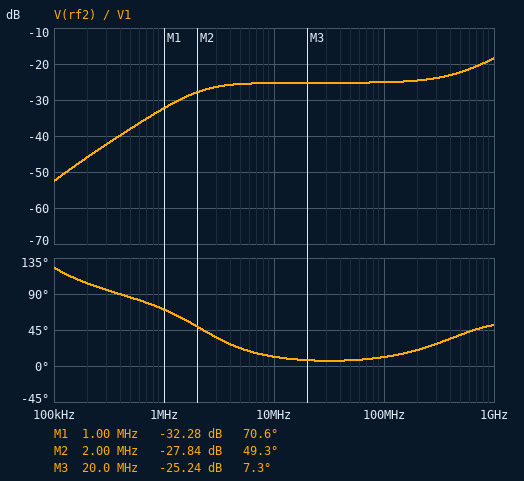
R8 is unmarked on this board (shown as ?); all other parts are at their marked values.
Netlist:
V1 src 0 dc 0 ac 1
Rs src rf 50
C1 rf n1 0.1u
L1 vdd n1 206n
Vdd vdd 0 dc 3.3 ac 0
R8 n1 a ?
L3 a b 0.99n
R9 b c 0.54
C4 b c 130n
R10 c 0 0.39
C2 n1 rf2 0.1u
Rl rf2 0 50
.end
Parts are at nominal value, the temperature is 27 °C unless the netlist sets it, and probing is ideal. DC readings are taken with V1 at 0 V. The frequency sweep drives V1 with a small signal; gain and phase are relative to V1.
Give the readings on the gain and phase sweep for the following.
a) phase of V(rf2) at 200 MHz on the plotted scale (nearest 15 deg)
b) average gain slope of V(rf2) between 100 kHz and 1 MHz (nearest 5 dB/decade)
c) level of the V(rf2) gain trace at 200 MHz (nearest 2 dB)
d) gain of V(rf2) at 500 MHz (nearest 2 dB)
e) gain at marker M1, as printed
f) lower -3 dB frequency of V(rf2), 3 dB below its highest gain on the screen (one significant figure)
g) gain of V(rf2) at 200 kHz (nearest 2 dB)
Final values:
15 deg
20 dB/decade
-24 dB
-22 dB
-32.28 dB
600 MHz
-46 dB
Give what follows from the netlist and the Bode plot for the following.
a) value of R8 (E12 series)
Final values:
2.7 Ω
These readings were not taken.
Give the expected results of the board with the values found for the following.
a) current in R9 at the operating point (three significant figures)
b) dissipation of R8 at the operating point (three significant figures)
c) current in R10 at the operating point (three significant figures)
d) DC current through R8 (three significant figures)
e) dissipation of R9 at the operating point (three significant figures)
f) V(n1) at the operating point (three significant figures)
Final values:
909 mA
2.23 W
909 mA
909 mA
446 mW
3.30 V
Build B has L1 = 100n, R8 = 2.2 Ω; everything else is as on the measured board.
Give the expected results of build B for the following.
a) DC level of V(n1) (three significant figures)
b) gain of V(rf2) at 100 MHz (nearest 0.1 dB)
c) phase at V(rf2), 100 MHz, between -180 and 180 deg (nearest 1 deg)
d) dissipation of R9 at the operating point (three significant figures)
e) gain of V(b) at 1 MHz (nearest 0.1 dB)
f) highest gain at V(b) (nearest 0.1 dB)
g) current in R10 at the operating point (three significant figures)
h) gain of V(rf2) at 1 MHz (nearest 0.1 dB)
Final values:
3.30 V
-26.4 dB
14 deg
600 mW
-49.1 dB
-42.3 dB
1.05 A
-38.1 dB
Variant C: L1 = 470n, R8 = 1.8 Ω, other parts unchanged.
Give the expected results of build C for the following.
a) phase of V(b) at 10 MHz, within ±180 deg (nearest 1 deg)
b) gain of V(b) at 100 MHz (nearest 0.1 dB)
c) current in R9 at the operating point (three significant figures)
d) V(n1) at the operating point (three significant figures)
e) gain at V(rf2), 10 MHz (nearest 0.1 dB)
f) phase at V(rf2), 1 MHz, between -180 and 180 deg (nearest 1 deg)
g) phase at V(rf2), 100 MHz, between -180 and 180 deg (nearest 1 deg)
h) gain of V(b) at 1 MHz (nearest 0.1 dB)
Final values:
-11 deg
-42.9 dB
1.21 A
3.30 V
-27.8 dB
40 deg
15 deg
-38.0 dB
